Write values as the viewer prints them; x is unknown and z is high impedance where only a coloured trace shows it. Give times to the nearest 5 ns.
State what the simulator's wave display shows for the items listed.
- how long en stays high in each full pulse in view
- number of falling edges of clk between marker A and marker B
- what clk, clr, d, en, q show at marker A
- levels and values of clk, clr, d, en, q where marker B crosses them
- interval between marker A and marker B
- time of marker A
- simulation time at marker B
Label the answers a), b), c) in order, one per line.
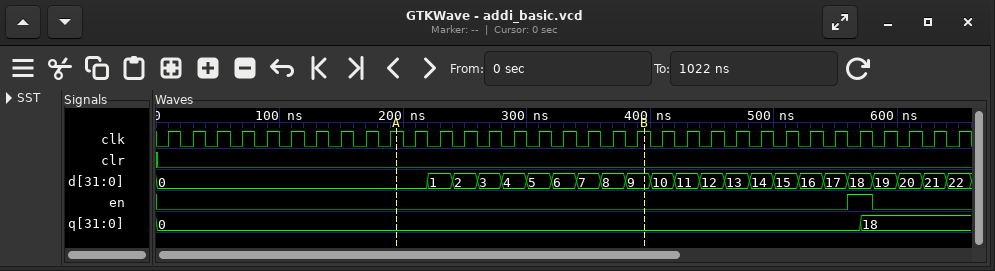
a) 20 ns
b) 10
c) clk=1, clr=0, d=0, en=0, q=0
d) clk=1, clr=0, d=9, en=0, q=0
e) 200 ns
f) 195 ns
g) 395 ns
